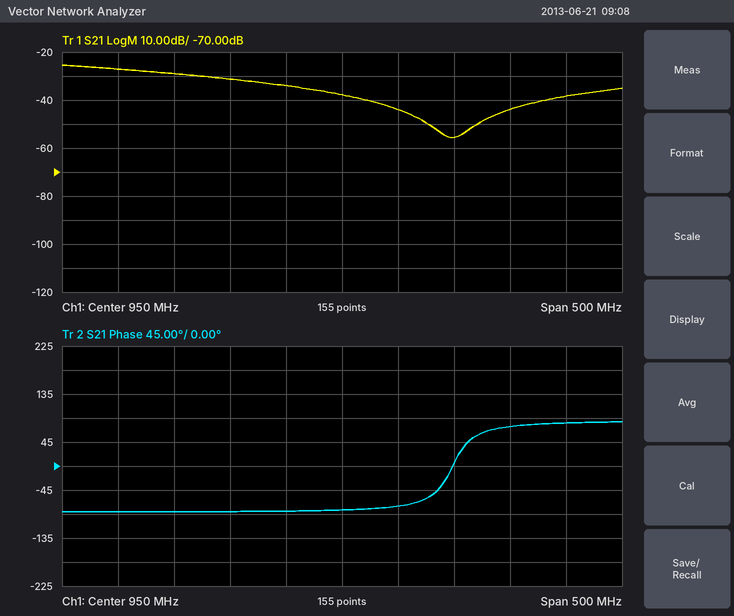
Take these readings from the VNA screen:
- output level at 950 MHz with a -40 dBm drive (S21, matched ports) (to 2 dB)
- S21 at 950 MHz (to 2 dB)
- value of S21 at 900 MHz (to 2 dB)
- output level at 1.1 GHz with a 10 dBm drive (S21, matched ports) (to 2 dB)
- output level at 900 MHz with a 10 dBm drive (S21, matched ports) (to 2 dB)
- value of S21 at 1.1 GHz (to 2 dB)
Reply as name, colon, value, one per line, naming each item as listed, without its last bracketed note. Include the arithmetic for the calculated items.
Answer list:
output level at 950 MHz with a -40 dBm drive (S21, matched ports): -40 dBm + (-38 dB) = -78 dBm
S21 at 950 MHz: -38 dB
value of S21 at 900 MHz: -34 dB
output level at 1.1 GHz with a 10 dBm drive (S21, matched ports): 10 dBm + (-44 dB) = -34 dBm
output level at 900 MHz with a 10 dBm drive (S21, matched ports): 10 dBm + (-34 dB) = -24 dBm
value of S21 at 1.1 GHz: -44 dB
